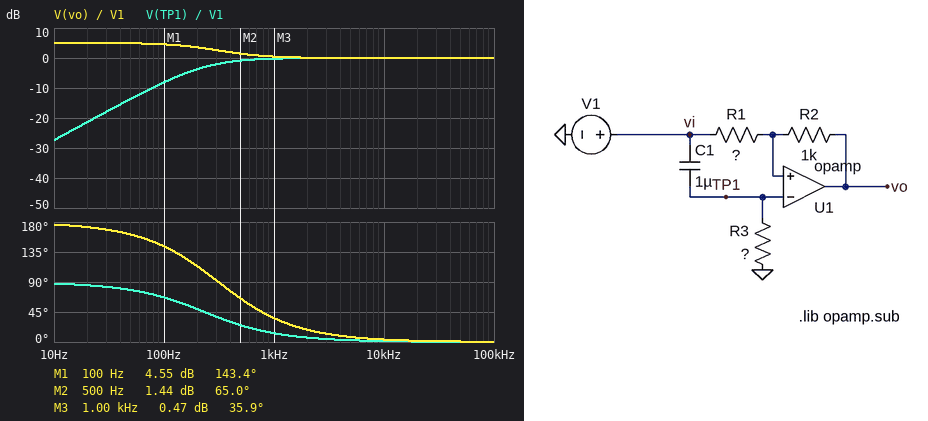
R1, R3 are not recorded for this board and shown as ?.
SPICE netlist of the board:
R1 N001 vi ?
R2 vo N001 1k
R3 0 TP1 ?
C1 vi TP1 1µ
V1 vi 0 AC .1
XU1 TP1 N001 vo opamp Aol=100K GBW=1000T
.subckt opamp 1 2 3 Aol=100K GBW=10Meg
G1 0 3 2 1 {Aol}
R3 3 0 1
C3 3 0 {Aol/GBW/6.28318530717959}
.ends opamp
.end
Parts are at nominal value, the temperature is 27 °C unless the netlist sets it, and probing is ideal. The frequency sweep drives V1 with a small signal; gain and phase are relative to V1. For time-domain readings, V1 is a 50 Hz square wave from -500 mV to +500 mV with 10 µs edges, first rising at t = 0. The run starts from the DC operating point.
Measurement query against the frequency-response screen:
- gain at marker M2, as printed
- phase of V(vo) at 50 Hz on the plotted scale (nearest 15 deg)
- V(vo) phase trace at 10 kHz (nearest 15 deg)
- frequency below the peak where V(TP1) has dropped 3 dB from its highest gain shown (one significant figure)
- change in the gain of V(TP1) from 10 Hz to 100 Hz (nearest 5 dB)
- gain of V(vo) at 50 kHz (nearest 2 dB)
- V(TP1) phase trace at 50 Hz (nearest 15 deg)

1.44 dB
165 deg
0 deg
200 Hz
20 dB
0 dB
75 deg
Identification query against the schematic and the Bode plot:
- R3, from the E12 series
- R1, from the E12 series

680 Ω
560 Ω
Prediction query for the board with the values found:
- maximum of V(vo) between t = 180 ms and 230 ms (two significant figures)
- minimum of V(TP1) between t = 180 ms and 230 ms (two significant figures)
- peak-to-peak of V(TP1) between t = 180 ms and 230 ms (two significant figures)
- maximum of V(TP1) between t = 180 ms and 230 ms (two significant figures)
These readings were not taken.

1.9 V
-990 mV
2.0 V
990 mV
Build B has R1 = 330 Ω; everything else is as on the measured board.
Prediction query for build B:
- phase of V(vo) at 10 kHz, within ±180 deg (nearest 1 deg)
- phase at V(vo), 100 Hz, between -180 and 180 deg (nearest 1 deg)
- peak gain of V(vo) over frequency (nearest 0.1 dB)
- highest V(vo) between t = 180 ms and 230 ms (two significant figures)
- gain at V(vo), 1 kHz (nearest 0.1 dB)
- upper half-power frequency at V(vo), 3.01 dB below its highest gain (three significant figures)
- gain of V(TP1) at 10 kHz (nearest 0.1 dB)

5 deg
149 deg
9.6 dB
2.5 V
1.5 dB
265 Hz
0 dB
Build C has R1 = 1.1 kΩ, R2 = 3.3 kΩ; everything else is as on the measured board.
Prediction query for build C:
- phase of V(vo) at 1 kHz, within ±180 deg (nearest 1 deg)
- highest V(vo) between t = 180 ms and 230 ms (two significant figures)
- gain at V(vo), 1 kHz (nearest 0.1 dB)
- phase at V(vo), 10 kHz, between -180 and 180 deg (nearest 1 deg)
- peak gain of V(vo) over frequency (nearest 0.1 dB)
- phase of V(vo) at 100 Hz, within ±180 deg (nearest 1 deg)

48 deg
2.5 V
1.5 dB
5 deg
9.5 dB
149 deg
